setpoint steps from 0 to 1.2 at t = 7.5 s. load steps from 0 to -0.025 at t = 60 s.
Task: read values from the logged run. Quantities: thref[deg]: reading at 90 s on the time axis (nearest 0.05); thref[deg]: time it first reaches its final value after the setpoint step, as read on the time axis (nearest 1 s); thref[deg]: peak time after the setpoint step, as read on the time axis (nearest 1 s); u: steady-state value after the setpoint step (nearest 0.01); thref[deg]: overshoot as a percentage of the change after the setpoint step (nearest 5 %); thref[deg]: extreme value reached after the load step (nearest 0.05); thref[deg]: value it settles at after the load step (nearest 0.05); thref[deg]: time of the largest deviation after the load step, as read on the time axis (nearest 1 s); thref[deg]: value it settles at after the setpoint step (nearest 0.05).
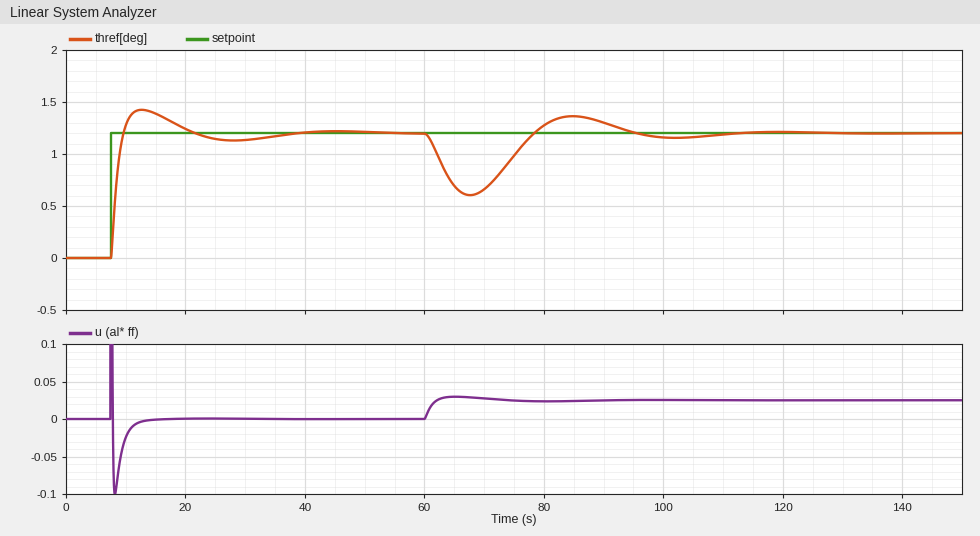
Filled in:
1.30
10 s
13 s
0.00
20 %
0.60
1.20
68 s
1.20
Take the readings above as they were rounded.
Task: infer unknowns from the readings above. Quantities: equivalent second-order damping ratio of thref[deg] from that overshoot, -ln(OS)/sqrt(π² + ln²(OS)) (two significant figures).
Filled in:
0.46
